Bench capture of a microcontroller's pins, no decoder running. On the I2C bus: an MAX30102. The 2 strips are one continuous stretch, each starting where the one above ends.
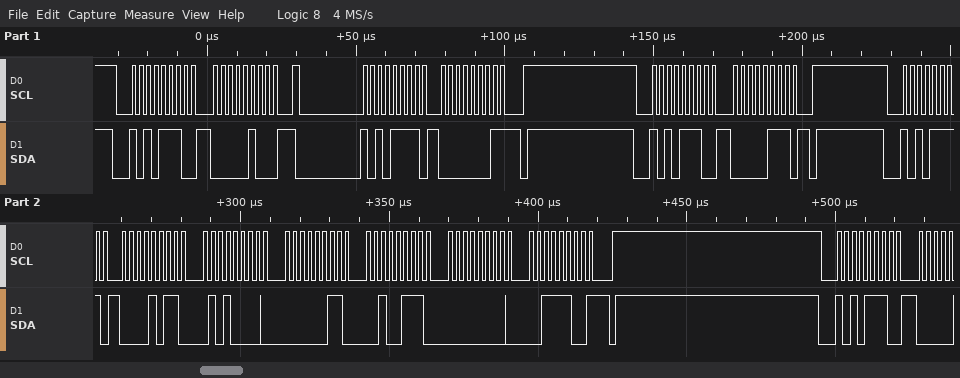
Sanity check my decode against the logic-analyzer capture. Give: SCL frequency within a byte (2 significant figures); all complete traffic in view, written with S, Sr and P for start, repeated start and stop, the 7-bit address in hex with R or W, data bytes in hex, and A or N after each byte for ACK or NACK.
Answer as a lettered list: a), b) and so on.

a) 400 kHz
b) S 57W A 04 A Sr 57R A 01 N P S 57W A 07 A P S 57R A 0B A 50 A 03 A 27 A 00 A 3C N P S 57W A
